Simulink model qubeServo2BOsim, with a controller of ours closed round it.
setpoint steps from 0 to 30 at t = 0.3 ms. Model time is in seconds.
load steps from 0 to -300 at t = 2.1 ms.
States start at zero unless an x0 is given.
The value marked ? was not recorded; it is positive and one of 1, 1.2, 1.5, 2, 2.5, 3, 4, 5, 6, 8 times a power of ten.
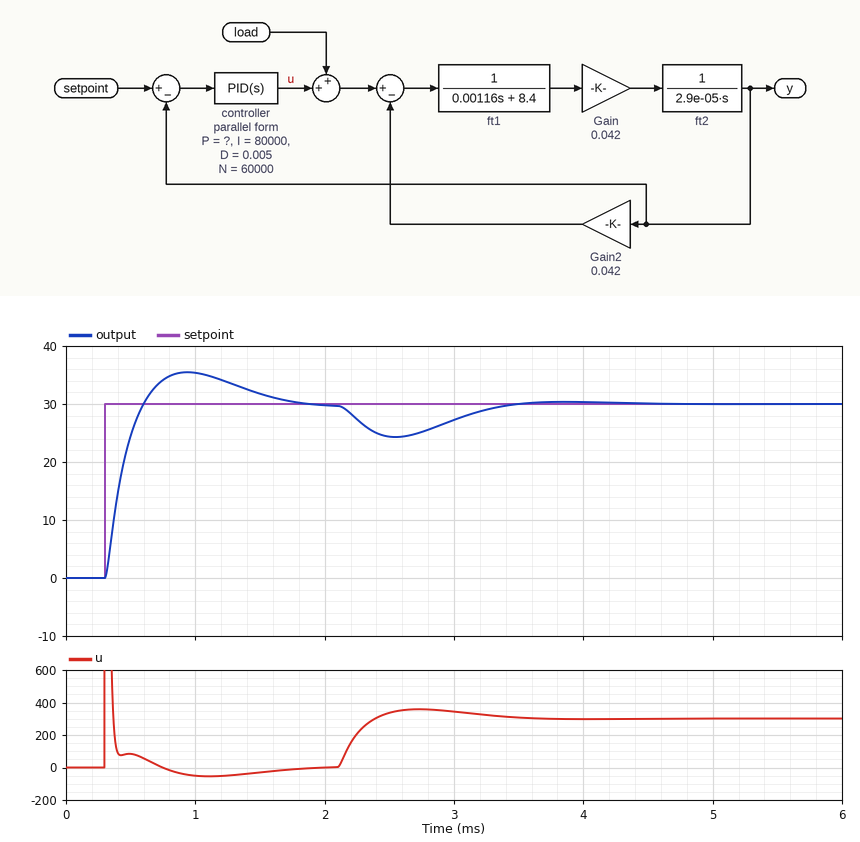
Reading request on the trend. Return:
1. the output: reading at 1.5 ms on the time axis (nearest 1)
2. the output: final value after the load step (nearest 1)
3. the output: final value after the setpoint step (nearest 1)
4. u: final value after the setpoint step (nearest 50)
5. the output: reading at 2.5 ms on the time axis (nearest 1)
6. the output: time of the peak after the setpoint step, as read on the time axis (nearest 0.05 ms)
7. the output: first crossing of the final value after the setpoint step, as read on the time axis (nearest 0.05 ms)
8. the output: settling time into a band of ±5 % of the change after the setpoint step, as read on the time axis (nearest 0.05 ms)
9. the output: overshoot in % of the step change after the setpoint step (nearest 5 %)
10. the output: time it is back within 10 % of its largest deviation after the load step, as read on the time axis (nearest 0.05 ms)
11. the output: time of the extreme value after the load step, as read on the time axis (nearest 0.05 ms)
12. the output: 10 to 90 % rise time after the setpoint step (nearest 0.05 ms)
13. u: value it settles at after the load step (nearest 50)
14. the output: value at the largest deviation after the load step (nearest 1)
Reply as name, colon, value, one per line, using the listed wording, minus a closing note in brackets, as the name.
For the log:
the output: reading at 1.5 ms on the time axis: 32
the output: final value after the load step: 30
the output: final value after the setpoint step: 30
u: final value after the setpoint step: 0
the output: reading at 2.5 ms on the time axis: 24
the output: time of the peak after the setpoint step, as read on the time axis: 0.95 ms
the output: first crossing of the final value after the setpoint step, as read on the time axis: 0.60 ms
the output: settling time into a band of ±5 % of the change after the setpoint step, as read on the time axis: 1.55 ms
the output: overshoot in % of the step change after the setpoint step: 20 %
the output: time it is back within 10 % of its largest deviation after the load step, as read on the time axis: 3.35 ms
the output: time of the extreme value after the load step, as read on the time axis: 2.55 ms
the output: 10 to 90 % rise time after the setpoint step: 0.20 ms
u: value it settles at after the load step: 300
the output: value at the largest deviation after the load step: 24
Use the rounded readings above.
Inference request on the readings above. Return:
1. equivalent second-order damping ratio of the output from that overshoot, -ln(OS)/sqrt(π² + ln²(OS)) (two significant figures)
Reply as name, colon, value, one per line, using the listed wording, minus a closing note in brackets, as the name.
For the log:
equivalent second-order damping ratio of the output from that overshoot, -ln(OS)/sqrt(π² + ln²(OS)): 0.46
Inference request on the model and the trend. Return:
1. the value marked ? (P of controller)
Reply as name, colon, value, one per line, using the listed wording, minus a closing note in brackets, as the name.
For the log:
the value marked ?: 40
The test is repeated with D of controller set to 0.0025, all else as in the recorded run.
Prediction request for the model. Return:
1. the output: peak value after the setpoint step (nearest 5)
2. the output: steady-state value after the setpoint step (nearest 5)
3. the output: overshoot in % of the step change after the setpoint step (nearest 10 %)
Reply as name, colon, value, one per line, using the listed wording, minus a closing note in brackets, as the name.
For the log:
the output: peak value after the setpoint step: 40
the output: steady-state value after the setpoint step: 30
the output: overshoot in % of the step change after the setpoint step: 30 %
